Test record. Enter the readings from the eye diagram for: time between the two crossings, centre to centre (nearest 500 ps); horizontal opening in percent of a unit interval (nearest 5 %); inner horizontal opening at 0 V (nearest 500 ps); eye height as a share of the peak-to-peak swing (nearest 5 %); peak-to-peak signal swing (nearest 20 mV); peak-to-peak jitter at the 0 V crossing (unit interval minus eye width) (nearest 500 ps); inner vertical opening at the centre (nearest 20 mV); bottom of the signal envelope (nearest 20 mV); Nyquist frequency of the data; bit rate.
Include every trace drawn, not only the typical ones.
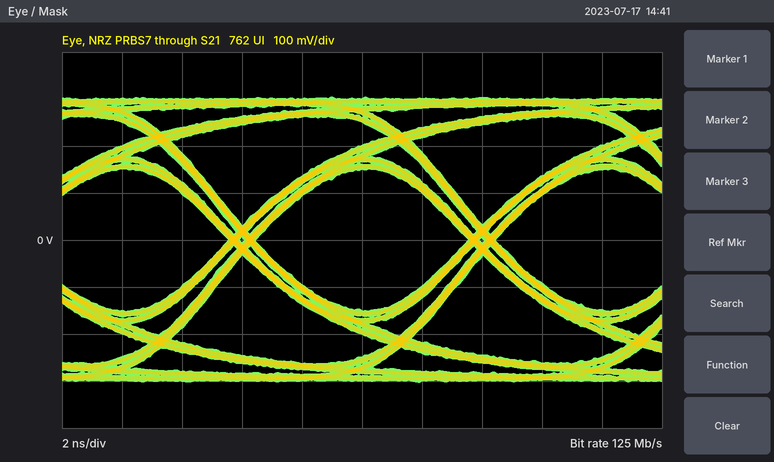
8.0 ns
90 %
7.0 ns
50 %
600 mV
1.0 ns
300 mV
-300 mV
62.5 MHz
125 Mb/s
